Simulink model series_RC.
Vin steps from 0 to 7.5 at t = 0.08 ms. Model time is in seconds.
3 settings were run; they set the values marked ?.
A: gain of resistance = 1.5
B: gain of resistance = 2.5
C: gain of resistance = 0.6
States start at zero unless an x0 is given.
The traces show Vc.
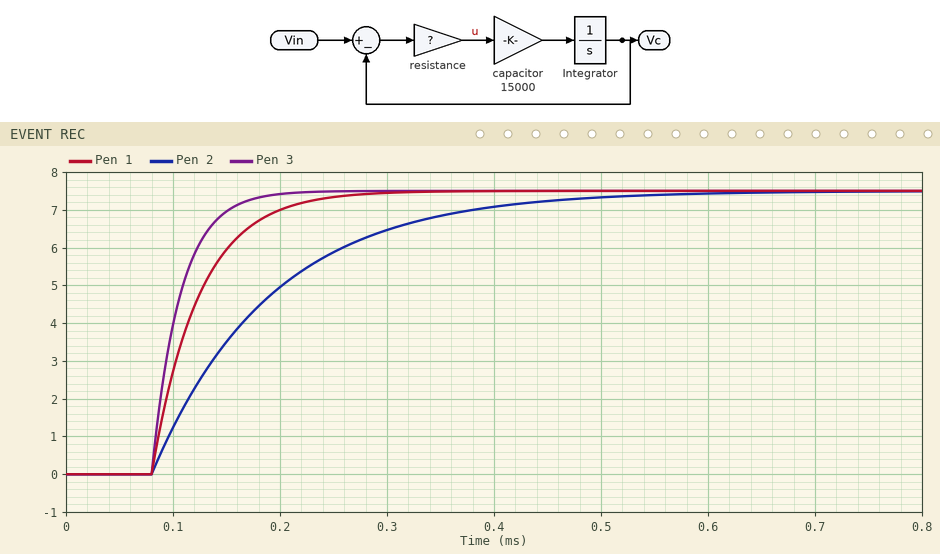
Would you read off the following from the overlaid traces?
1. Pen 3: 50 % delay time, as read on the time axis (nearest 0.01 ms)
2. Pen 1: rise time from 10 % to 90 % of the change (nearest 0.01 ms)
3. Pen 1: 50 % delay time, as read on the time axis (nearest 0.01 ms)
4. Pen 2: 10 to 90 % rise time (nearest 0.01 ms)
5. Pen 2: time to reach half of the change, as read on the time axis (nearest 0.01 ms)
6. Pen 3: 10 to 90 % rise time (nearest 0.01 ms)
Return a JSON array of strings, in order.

["0.10 ms", "0.10 ms", "0.11 ms", "0.24 ms", "0.16 ms", "0.06 ms"]
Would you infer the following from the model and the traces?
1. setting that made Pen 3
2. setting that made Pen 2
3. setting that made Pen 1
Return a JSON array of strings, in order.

["B", "C", "A"]
